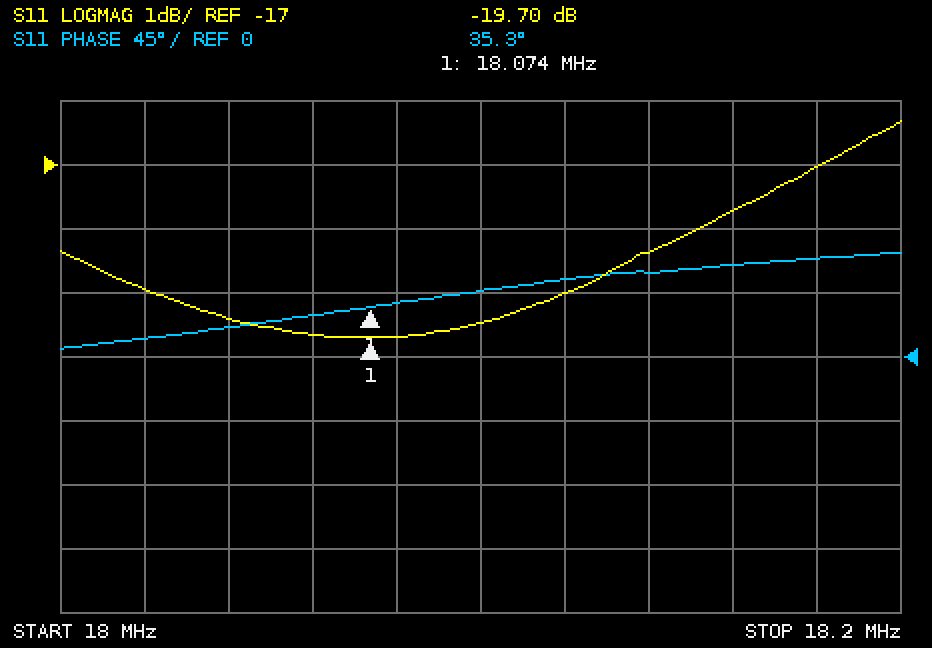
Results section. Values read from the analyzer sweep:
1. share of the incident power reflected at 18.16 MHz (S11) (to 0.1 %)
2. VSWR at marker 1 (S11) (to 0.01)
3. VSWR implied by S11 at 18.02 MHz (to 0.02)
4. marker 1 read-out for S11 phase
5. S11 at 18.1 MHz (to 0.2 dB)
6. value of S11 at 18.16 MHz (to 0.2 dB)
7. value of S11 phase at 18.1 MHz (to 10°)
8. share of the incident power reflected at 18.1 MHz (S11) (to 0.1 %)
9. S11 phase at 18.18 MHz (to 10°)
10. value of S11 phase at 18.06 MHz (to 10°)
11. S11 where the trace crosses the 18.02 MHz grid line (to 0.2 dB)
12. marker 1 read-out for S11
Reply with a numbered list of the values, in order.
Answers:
1. 1.7 %
2. 1.23
3. 1.26
4. 35.3°
5. -19.4 dB
6. -17.8 dB
7. 50°
8. 1.1 %
9. 70°
10. 30°
11. -19.0 dB
12. -19.70 dB
